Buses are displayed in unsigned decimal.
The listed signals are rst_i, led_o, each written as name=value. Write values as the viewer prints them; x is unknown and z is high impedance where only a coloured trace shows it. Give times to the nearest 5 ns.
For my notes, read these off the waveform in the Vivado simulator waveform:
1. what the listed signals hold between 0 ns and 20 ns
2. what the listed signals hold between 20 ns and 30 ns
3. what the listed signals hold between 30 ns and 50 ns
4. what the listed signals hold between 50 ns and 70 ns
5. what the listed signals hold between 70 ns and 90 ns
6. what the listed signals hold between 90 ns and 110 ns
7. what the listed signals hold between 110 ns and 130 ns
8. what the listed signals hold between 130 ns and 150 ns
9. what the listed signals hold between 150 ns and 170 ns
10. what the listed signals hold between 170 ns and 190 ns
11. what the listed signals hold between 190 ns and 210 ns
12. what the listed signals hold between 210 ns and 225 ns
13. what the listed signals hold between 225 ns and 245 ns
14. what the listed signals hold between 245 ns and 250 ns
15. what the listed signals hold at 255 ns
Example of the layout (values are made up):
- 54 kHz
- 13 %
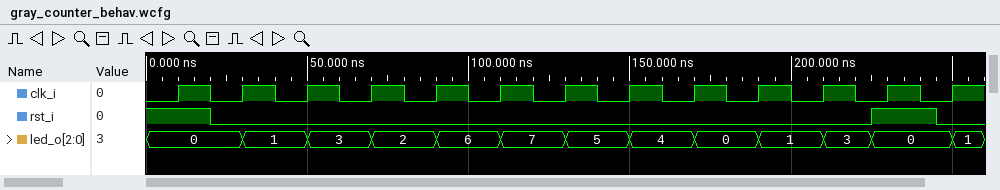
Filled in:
- rst_i=1, led_o=0
- rst_i=0, led_o=0
- rst_i=0, led_o=1
- rst_i=0, led_o=3
- rst_i=0, led_o=2
- rst_i=0, led_o=6
- rst_i=0, led_o=7
- rst_i=0, led_o=5
- rst_i=0, led_o=4
- rst_i=0, led_o=0
- rst_i=0, led_o=1
- rst_i=0, led_o=3
- rst_i=1, led_o=0
- rst_i=0, led_o=0
- rst_i=0, led_o=1
